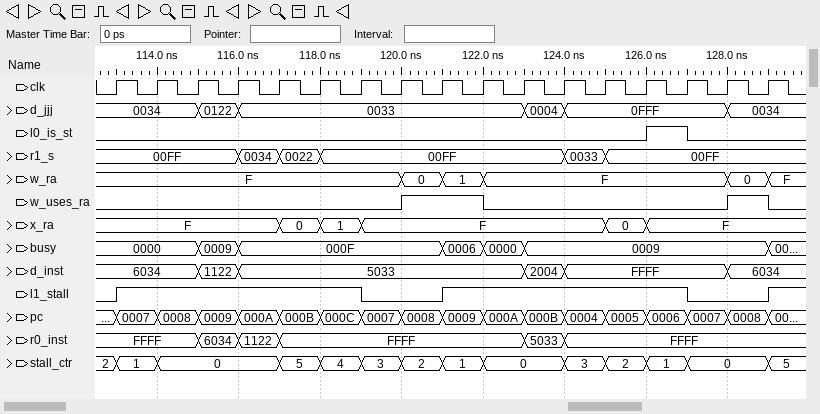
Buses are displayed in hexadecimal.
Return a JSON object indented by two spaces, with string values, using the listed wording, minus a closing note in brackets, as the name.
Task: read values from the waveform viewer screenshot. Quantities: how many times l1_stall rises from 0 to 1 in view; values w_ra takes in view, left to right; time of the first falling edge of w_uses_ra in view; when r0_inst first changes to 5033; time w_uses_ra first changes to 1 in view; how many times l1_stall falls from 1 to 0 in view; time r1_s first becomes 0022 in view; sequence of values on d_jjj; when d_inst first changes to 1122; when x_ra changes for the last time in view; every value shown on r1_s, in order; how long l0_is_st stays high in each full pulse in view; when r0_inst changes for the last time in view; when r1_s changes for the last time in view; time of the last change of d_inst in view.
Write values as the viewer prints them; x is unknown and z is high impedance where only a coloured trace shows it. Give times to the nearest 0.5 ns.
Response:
{
  "how many times l1_stall rises from 0 to 1 in view": "3",
  "values w_ra takes in view, left to right": "F, 0, 1, F, 0, F",
  "time of the first falling edge of w_uses_ra in view": "122 ns",
  "when r0_inst first changes to 5033": "123 ns",
  "time w_uses_ra first changes to 1 in view": "120 ns",
  "how many times l1_stall falls from 1 to 0 in view": "2",
  "time r1_s first becomes 0022 in view": "117 ns",
  "sequence of values on d_jjj": "0034, 0122, 0033, 0004, 0FFF, 0034",
  "when d_inst first changes to 1122": "115 ns",
  "when x_ra changes for the last time in view": "126 ns",
  "every value shown on r1_s, in order": "00FF, 0034, 0022, 00FF, 0033, 00FF",
  "how long l0_is_st stays high in each full pulse in view": "1 ns",
  "when r0_inst changes for the last time in view": "124 ns",
  "when r1_s changes for the last time in view": "125 ns",
  "time of the last change of d_inst in view": "128 ns"
}
